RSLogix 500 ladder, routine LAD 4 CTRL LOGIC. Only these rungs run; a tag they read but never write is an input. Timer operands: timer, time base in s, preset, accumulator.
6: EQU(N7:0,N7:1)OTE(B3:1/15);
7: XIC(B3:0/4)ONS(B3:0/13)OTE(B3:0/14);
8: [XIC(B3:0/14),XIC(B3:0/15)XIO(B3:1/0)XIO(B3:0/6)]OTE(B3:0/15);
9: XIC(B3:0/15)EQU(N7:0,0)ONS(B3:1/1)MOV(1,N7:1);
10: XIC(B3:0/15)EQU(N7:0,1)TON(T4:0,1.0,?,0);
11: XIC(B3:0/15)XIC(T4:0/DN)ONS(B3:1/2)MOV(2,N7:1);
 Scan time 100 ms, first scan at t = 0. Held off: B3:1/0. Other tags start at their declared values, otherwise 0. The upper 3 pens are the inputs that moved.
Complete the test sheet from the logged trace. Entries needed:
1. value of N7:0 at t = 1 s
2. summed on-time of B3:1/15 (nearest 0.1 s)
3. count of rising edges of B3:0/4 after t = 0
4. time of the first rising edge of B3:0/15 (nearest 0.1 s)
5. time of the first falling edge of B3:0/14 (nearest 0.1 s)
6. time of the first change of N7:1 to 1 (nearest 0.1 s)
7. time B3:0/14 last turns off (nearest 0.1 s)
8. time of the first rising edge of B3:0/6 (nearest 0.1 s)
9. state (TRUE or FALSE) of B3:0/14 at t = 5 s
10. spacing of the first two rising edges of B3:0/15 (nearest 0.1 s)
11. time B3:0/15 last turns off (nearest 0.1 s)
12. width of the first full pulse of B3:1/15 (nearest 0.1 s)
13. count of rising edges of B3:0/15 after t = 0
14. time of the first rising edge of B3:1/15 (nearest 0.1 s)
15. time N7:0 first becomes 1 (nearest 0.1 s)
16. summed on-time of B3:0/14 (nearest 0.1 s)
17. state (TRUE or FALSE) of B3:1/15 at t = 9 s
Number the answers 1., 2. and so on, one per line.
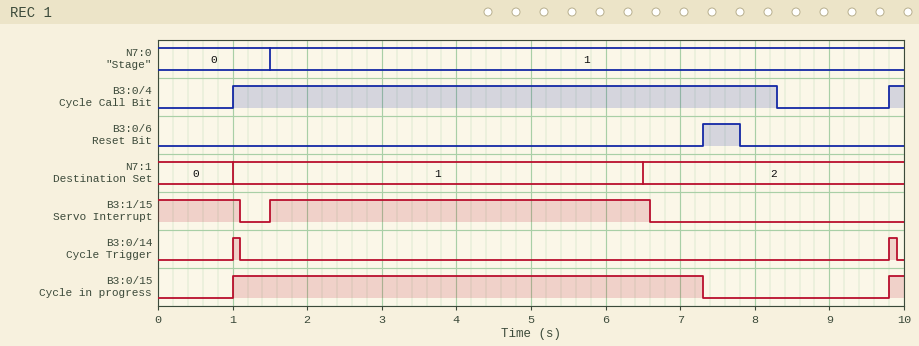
1. 0
2. 6.2 s
3. 2
4. 1.0 s
5. 1.1 s
6. 1.0 s
7. 9.9 s
8. 7.3 s
9. FALSE
10. 8.8 s
11. 7.3 s
12. 5.1 s
13. 2
14. 1.5 s
15. 1.5 s
16. 0.2 s
17. FALSE
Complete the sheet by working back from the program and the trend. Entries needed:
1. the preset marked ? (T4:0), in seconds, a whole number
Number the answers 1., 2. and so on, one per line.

1. 5 s
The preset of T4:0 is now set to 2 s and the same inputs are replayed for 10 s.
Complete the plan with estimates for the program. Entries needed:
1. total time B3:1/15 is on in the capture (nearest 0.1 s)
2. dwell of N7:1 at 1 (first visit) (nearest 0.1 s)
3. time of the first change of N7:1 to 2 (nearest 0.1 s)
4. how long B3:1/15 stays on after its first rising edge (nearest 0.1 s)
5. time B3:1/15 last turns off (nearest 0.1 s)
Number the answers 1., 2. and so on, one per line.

1. 3.2 s
2. 2.5 s
3. 3.5 s
4. 2.1 s
5. 3.6 s
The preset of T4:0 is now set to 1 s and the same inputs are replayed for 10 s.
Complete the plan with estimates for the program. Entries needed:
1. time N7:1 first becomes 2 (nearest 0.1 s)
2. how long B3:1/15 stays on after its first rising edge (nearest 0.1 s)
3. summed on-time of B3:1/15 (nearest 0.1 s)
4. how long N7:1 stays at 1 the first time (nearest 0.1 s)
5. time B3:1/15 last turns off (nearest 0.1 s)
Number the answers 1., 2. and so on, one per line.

1. 2.5 s
2. 1.1 s
3. 2.2 s
4. 1.5 s
5. 2.6 s
